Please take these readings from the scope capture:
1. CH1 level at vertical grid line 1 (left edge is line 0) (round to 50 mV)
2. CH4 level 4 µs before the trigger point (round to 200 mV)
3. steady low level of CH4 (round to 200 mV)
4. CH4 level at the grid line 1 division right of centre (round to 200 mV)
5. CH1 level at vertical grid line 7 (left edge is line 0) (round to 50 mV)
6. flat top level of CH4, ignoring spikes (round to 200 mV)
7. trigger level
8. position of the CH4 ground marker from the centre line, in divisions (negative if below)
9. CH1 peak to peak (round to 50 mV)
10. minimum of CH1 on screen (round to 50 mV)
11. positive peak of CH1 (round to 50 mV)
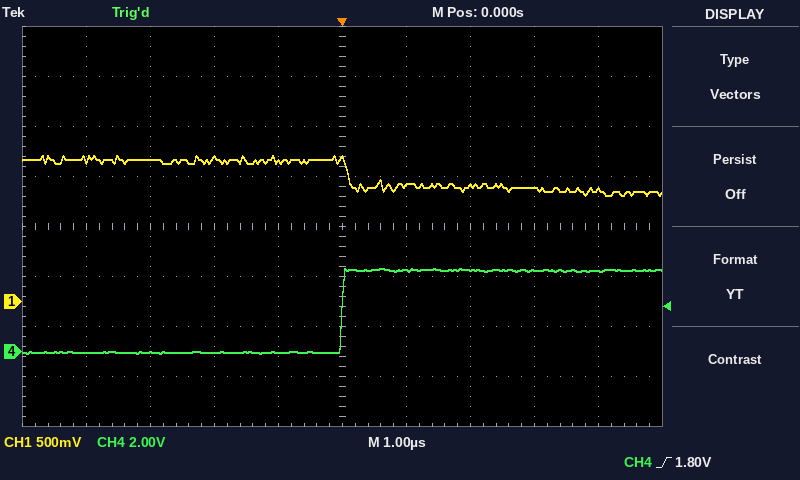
1.40 V
0.0 V
0.0 V
3.2 V
1.15 V
3.2 V
1.80 V
-2.5 div
400 mV
1.05 V
1.45 V
